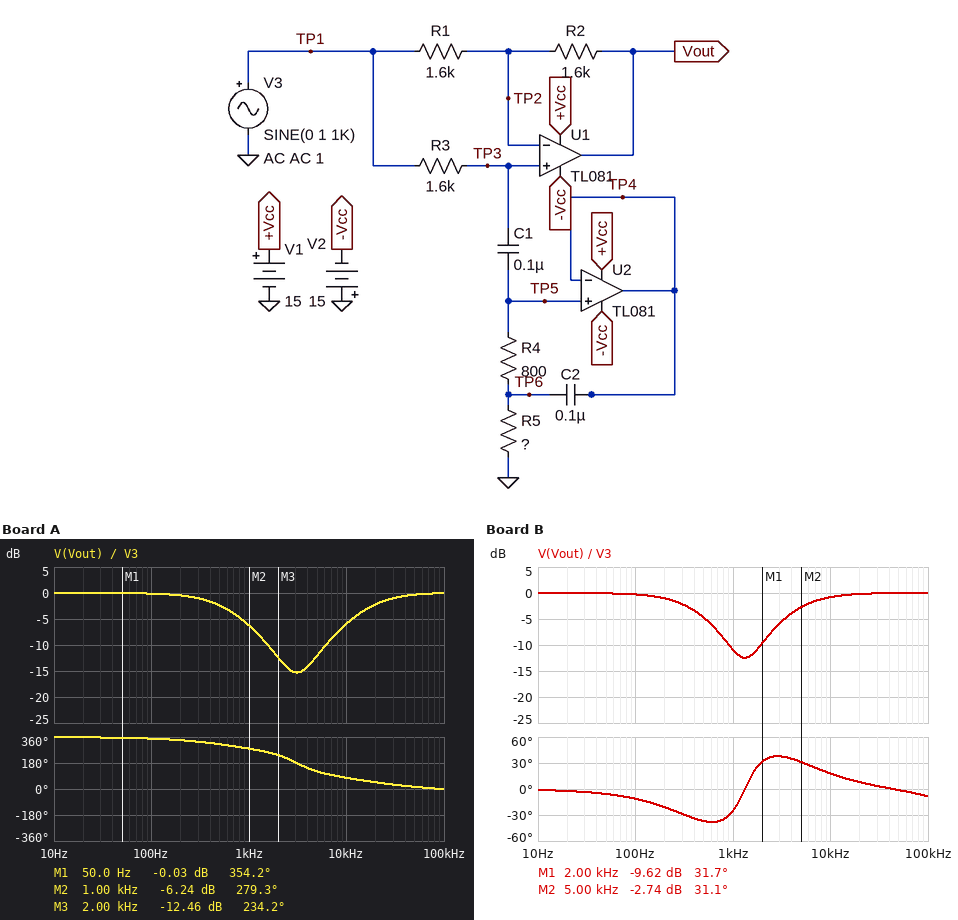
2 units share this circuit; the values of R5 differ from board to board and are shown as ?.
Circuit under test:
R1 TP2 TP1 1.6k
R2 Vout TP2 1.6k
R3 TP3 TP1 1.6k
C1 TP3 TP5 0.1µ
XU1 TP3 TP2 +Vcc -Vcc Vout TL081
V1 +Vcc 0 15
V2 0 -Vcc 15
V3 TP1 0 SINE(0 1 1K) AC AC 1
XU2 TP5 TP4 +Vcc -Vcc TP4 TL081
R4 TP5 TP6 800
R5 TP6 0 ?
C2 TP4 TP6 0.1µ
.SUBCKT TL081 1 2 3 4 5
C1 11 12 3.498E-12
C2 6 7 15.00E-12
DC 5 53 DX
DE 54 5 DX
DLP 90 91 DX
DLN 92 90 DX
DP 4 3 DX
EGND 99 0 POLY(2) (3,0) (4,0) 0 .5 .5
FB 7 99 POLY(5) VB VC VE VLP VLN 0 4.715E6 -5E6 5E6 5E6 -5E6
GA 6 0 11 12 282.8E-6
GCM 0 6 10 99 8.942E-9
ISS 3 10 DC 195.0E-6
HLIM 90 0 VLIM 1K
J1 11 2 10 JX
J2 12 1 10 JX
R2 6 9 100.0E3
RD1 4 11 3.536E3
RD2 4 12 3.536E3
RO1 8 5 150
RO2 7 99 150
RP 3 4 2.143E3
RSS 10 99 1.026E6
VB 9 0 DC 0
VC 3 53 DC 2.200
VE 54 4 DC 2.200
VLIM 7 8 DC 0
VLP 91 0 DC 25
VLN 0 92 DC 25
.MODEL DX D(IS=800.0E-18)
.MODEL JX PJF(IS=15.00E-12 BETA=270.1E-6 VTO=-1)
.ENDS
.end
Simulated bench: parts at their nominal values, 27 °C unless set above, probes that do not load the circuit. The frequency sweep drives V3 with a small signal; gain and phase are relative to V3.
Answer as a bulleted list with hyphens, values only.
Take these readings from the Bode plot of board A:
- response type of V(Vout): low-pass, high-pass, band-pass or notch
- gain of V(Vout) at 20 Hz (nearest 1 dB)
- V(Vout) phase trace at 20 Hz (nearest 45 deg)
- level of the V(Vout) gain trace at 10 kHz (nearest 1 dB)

- notch
- 0 dB
- 360 deg
- -6 dB
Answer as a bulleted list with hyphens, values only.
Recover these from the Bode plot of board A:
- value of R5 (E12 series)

- 330 Ω
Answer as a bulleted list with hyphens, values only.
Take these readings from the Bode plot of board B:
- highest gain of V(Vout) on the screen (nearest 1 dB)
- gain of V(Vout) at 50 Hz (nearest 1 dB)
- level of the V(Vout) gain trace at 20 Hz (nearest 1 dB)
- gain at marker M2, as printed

- 0 dB
- 0 dB
- 0 dB
- -2.74 dB
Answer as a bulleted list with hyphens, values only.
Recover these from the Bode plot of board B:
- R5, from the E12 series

- 1.8 kΩ
